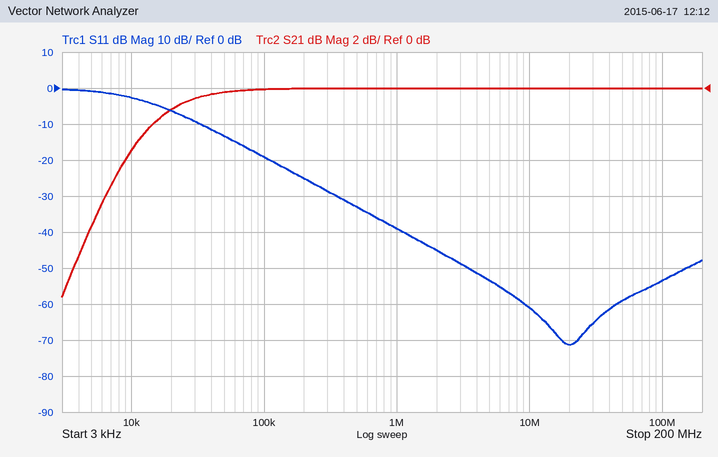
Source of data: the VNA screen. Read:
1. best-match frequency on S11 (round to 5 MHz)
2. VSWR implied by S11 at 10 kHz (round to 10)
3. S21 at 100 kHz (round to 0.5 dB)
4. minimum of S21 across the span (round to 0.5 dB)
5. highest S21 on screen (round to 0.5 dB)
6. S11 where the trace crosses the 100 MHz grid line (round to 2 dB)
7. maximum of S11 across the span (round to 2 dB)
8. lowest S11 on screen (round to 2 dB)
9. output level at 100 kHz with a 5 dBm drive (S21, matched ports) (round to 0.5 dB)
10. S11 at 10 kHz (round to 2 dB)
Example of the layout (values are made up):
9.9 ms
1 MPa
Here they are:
20 MHz
10
0.0 dB
-11.5 dB
0.0 dB
-54 dB
0 dB
-72 dB
5.0 dBm
-2 dB
